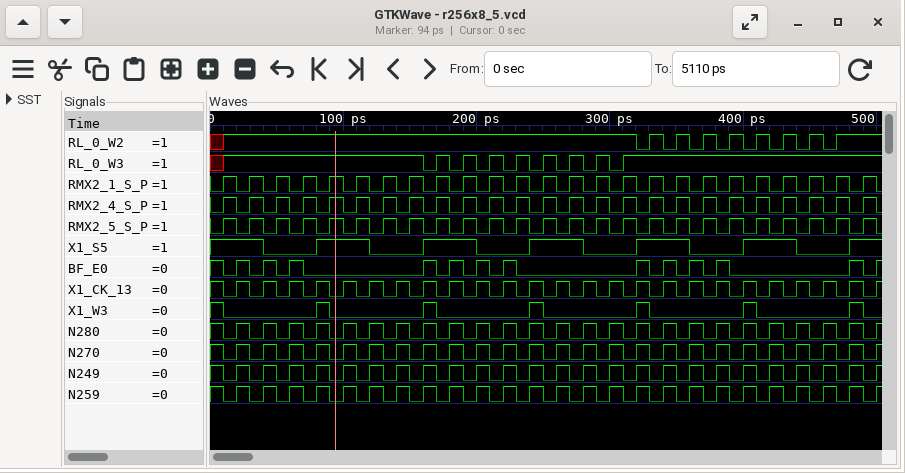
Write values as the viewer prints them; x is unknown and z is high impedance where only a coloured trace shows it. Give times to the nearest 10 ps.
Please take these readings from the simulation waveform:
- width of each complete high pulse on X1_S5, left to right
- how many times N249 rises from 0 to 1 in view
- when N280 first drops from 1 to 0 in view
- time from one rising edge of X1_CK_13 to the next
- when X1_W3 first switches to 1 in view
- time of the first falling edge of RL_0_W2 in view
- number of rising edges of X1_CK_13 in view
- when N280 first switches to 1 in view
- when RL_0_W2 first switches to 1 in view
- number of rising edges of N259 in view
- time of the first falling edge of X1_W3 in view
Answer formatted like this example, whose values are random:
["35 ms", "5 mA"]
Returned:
["40 ps, 40 ps, 40 ps, 40 ps, 40 ps", "25", "10 ps", "20 ps", "80 ps", "320 ps", "25", "20 ps", "10 ps", "25", "10 ps"]
